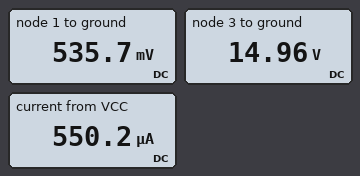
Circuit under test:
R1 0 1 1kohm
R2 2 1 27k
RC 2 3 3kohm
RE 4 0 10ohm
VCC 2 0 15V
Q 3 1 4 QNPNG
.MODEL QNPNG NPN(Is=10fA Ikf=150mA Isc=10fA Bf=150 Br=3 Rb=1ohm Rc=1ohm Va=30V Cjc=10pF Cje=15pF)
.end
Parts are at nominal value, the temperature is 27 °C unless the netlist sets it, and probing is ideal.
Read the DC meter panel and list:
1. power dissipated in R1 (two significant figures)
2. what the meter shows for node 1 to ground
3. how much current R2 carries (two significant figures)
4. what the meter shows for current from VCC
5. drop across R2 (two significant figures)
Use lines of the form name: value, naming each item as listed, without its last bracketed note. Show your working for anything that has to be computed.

power dissipated in R1: (535.7 mV)^2 / 1 kΩ = 290 µW
what the meter shows for node 1 to ground: 535.7 mV
how much current R2 carries: (15 V - 535.7 mV) / 27 kΩ = 540 µA
what the meter shows for current from VCC: 550.2 µA
drop across R2: 15 V - 535.7 mV = 14 V
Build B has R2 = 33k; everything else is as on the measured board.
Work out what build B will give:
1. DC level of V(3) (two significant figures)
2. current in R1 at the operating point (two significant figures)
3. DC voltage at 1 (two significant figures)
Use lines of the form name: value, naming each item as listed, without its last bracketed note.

DC level of V(3): 15 V
current in R1 at the operating point: 440 µA
DC voltage at 1: 440 mV
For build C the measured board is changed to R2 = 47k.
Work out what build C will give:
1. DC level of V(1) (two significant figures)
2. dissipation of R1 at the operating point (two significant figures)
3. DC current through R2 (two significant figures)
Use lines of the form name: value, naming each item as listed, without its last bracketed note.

DC level of V(1): 310 mV
dissipation of R1 at the operating point: 98 µW
DC current through R2: 310 µA
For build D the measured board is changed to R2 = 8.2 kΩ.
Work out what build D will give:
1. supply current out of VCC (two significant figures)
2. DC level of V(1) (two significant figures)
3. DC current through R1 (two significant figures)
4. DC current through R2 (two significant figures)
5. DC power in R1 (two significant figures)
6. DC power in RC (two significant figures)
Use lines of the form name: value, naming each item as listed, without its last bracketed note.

supply current out of VCC: 6.7 mA
DC level of V(1): 770 mV
DC current through R1: 770 µA
DC current through R2: 1.7 mA
DC power in R1: 600 µW
DC power in RC: 74 mW
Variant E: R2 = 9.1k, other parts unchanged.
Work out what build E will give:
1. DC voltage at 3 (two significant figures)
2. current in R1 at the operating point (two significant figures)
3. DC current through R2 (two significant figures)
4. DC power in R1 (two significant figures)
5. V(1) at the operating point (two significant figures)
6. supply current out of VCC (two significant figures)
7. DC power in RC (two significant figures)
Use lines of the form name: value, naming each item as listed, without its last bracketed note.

DC voltage at 3: 97 mV
current in R1 at the operating point: 770 µA
DC current through R2: 1.6 mA
DC power in R1: 590 µW
V(1) at the operating point: 770 mV
supply current out of VCC: 6.5 mA
DC power in RC: 74 mW
